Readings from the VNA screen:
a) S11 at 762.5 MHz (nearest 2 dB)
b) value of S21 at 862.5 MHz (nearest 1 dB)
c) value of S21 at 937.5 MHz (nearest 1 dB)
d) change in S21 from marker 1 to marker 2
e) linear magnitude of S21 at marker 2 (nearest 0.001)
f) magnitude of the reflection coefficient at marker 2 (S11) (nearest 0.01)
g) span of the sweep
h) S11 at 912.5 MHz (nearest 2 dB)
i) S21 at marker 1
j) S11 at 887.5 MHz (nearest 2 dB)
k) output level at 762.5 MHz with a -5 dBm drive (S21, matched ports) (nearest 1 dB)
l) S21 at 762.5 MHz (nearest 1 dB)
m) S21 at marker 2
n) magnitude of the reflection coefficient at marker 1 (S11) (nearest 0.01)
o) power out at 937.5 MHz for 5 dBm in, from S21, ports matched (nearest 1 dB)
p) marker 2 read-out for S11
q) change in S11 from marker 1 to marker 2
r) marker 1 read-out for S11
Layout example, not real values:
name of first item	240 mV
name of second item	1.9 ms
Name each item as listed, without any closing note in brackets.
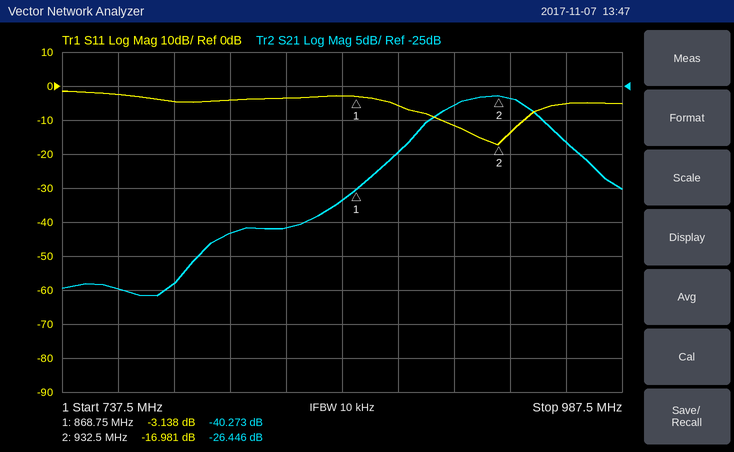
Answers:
S11 at 762.5 MHz	-2 dB
value of S21 at 862.5 MHz	-42 dB
value of S21 at 937.5 MHz	-27 dB
change in S21 from marker 1 to marker 2	13.827 dB
linear magnitude of S21 at marker 2	0.048
magnitude of the reflection coefficient at marker 2 (S11)	0.14
span of the sweep	250 MHz
S11 at 912.5 MHz	-12 dB
S21 at marker 1	-40.273 dB
S11 at 887.5 MHz	-6 dB
output level at 762.5 MHz with a -5 dBm drive (S21, matched ports)	-60 dBm
S21 at 762.5 MHz	-55 dB
S21 at marker 2	-26.446 dB
magnitude of the reflection coefficient at marker 1 (S11)	0.70
power out at 937.5 MHz for 5 dBm in, from S21, ports matched	-22 dBm
marker 2 read-out for S11	-16.981 dB
change in S11 from marker 1 to marker 2	-13.843 dB
marker 1 read-out for S11	-3.138 dB
